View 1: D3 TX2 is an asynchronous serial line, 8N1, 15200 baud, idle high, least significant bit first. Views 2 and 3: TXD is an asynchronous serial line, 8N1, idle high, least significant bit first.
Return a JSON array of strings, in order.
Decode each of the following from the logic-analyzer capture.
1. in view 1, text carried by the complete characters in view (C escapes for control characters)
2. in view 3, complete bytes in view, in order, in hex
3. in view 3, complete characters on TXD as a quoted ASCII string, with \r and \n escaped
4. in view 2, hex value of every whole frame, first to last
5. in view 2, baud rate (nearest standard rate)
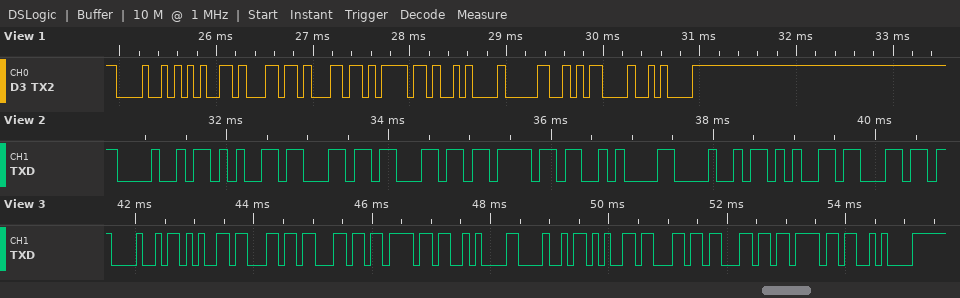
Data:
["\"Hello\\n0\\r\\n\"", "48 65 6C 6C 6F 0A 48 65 6C 6C 6F 0A", "\"Hello\\nHello\\n\"", "0x48 0x65 0x6C 0x6C 0x6F 0x0A 0x48 0x65 0x6C", "9600 baud"]
